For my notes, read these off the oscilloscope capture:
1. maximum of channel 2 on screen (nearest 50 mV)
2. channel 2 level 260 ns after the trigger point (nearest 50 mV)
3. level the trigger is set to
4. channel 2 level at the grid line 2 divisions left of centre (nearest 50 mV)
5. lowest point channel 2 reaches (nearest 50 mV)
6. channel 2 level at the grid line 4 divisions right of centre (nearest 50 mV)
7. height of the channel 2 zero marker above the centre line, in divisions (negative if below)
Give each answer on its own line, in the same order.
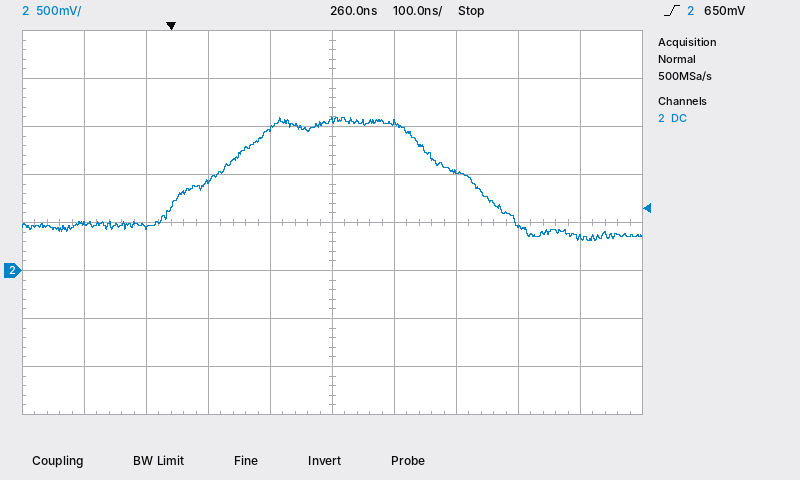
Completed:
1.60 V
1.55 V
650 mV
950 mV
300 mV
350 mV
-1.0 div
